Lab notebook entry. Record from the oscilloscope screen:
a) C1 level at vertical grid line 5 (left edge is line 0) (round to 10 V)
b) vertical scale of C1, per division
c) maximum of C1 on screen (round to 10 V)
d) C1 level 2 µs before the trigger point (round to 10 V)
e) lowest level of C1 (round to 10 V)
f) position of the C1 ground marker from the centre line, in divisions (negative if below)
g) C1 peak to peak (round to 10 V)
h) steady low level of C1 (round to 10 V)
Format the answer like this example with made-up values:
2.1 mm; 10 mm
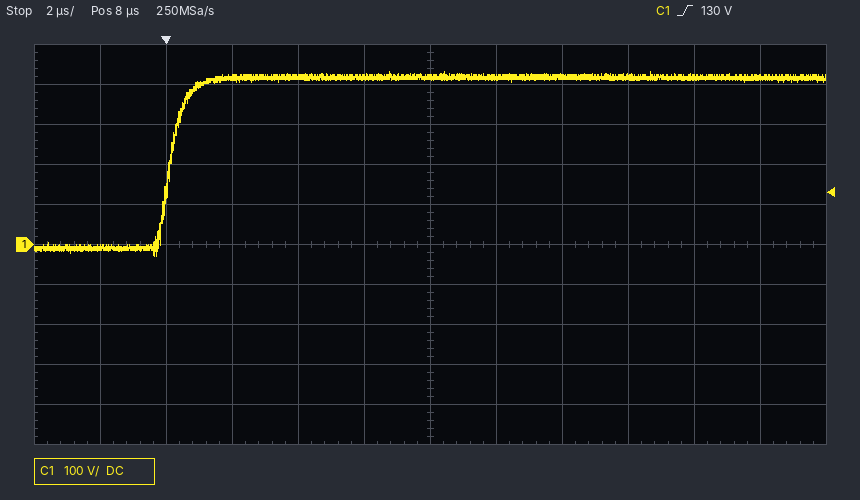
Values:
420 V; 100 V; 430 V; -10 V; -30 V; 0.0 div; 460 V; -10 V
